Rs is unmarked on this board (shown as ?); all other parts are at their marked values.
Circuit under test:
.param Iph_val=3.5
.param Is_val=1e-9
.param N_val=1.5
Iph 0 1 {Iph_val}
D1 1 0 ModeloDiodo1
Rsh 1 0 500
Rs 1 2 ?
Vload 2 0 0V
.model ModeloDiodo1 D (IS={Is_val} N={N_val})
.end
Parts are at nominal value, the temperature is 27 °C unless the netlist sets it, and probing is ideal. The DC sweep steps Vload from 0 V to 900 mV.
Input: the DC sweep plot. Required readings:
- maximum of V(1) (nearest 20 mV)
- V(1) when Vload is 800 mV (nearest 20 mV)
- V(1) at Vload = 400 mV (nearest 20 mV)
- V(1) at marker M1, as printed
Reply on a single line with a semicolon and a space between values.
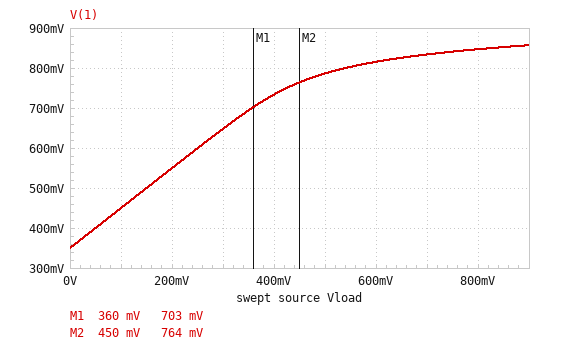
860 mV; 840 mV; 740 mV; 703 mV
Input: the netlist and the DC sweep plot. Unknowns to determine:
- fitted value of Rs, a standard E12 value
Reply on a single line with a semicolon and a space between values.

0.1 Ω
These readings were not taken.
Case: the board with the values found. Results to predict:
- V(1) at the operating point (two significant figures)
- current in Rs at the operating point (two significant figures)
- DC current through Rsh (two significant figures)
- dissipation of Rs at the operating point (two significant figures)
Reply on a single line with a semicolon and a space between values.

350 mV; 3.5 A; 700 µA; 1.2 W
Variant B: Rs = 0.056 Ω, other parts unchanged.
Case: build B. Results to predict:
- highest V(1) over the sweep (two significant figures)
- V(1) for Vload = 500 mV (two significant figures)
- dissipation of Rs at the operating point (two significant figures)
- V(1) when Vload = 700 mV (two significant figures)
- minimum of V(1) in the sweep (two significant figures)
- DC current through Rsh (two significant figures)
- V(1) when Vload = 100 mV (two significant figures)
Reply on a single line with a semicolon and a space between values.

860 mV; 690 mV; 690 mW; 820 mV; 200 mV; 390 µA; 300 mV
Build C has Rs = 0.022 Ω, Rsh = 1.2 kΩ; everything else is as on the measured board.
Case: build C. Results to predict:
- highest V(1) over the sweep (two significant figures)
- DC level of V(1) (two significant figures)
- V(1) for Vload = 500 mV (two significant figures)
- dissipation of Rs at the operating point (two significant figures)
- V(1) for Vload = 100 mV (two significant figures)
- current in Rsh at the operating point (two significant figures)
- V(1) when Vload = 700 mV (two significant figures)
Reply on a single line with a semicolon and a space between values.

870 mV; 77 mV; 580 mV; 270 mW; 180 mV; 64 µA; 770 mV
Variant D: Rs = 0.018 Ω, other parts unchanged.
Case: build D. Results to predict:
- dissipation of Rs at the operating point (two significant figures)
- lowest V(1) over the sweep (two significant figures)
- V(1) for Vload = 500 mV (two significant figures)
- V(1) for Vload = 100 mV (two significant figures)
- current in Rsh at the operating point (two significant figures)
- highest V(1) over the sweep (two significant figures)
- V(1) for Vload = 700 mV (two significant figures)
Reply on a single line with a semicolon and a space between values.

220 mW; 63 mV; 560 mV; 160 mV; 130 µA; 870 mV; 760 mV
